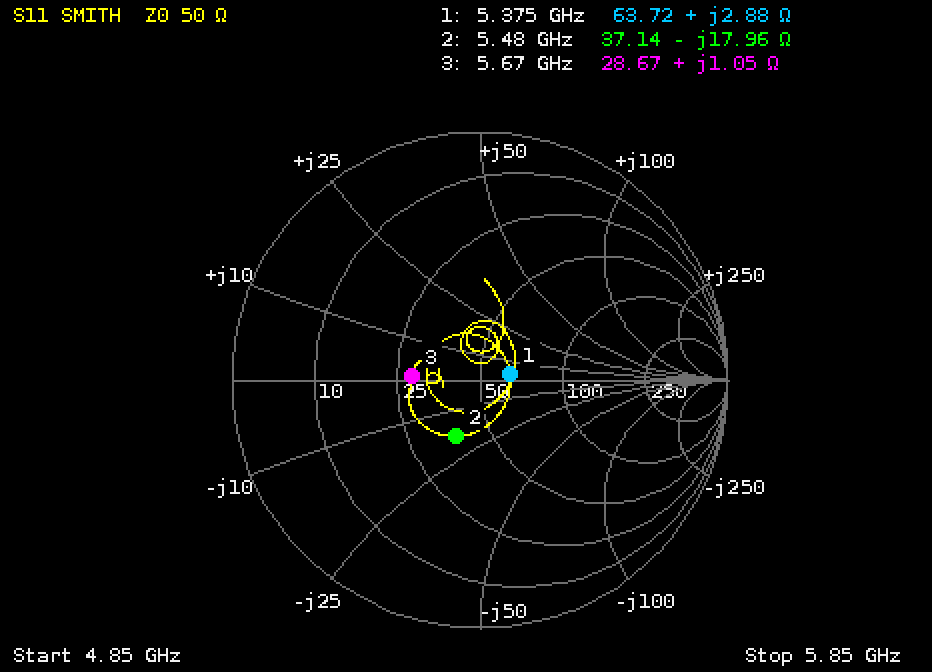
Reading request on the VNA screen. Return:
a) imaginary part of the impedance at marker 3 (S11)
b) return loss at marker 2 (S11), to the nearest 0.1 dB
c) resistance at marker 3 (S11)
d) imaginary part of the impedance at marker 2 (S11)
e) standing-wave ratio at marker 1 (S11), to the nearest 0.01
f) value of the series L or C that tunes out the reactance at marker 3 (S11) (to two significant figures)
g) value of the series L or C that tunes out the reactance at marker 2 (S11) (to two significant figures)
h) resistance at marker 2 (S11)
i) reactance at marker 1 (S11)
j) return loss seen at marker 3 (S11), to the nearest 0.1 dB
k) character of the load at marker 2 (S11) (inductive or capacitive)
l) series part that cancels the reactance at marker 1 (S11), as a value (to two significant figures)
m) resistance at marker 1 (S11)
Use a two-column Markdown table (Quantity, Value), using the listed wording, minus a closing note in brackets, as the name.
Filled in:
| Quantity | Value |
|---|---|
| imaginary part of the impedance at marker 3 | +1.05 Ω |
| return loss at marker 2 (S11), to the nearest 0.1 dB | 12.1 dB |
| resistance at marker 3 | 28.67 Ω |
| imaginary part of the impedance at marker 2 | -17.96 Ω |
| standing-wave ratio at marker 1 (S11), to the nearest 0.01 | 1.28 |
| value of the series L or C that tunes out the reactance at marker 3 (S11) | 27 pF |
| value of the series L or C that tunes out the reactance at marker 2 (S11) | 520 pH |
| resistance at marker 2 | 37.14 Ω |
| reactance at marker 1 | +2.88 Ω |
| return loss seen at marker 3 (S11), to the nearest 0.1 dB | 11.3 dB |
| character of the load at marker 2 (S11) | capacitive |
| series part that cancels the reactance at marker 1 (S11), as a value | 10 pF |
| resistance at marker 1 | 63.72 Ω |
